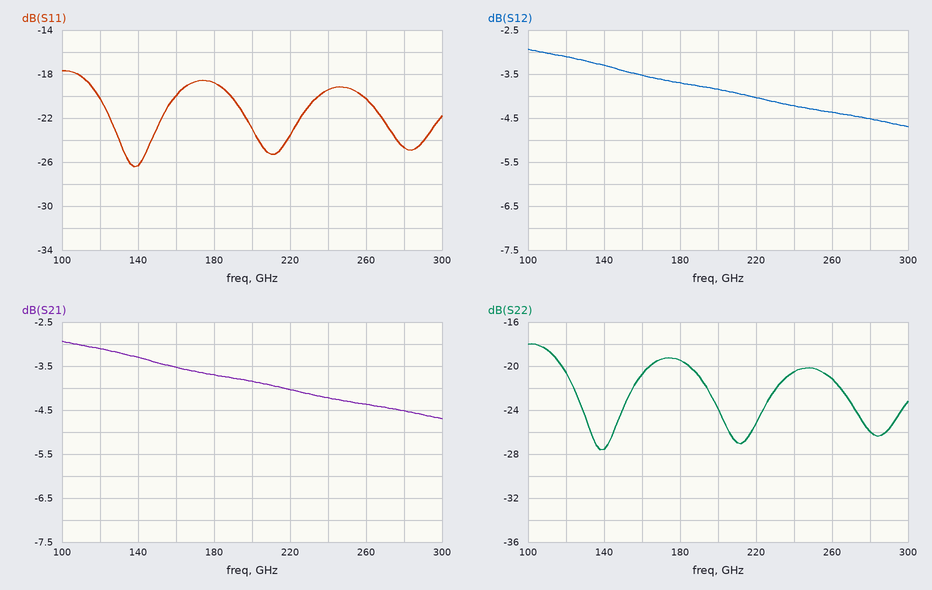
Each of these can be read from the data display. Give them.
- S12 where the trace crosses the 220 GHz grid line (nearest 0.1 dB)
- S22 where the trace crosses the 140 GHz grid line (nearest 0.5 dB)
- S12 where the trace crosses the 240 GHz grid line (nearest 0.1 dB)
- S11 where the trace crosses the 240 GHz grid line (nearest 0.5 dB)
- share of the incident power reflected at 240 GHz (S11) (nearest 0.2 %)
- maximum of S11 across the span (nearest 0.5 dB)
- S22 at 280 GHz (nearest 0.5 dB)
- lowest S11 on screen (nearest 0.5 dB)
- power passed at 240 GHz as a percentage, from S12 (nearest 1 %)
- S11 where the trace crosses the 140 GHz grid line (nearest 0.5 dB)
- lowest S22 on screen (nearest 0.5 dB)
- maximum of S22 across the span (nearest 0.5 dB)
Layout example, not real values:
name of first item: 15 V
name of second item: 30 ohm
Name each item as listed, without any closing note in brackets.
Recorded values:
S12 where the trace crosses the 220 GHz grid line: -4.0 dB
S22 where the trace crosses the 140 GHz grid line: -27.5 dB
S12 where the trace crosses the 240 GHz grid line: -4.2 dB
S11 where the trace crosses the 240 GHz grid line: -19.5 dB
share of the incident power reflected at 240 GHz (S11): 1.2 %
maximum of S11 across the span: -17.5 dB
S22 at 280 GHz: -26.0 dB
lowest S11 on screen: -26.5 dB
power passed at 240 GHz as a percentage, from S12: 38 %
S11 where the trace crosses the 140 GHz grid line: -26.5 dB
lowest S22 on screen: -27.5 dB
maximum of S22 across the span: -18.0 dB
